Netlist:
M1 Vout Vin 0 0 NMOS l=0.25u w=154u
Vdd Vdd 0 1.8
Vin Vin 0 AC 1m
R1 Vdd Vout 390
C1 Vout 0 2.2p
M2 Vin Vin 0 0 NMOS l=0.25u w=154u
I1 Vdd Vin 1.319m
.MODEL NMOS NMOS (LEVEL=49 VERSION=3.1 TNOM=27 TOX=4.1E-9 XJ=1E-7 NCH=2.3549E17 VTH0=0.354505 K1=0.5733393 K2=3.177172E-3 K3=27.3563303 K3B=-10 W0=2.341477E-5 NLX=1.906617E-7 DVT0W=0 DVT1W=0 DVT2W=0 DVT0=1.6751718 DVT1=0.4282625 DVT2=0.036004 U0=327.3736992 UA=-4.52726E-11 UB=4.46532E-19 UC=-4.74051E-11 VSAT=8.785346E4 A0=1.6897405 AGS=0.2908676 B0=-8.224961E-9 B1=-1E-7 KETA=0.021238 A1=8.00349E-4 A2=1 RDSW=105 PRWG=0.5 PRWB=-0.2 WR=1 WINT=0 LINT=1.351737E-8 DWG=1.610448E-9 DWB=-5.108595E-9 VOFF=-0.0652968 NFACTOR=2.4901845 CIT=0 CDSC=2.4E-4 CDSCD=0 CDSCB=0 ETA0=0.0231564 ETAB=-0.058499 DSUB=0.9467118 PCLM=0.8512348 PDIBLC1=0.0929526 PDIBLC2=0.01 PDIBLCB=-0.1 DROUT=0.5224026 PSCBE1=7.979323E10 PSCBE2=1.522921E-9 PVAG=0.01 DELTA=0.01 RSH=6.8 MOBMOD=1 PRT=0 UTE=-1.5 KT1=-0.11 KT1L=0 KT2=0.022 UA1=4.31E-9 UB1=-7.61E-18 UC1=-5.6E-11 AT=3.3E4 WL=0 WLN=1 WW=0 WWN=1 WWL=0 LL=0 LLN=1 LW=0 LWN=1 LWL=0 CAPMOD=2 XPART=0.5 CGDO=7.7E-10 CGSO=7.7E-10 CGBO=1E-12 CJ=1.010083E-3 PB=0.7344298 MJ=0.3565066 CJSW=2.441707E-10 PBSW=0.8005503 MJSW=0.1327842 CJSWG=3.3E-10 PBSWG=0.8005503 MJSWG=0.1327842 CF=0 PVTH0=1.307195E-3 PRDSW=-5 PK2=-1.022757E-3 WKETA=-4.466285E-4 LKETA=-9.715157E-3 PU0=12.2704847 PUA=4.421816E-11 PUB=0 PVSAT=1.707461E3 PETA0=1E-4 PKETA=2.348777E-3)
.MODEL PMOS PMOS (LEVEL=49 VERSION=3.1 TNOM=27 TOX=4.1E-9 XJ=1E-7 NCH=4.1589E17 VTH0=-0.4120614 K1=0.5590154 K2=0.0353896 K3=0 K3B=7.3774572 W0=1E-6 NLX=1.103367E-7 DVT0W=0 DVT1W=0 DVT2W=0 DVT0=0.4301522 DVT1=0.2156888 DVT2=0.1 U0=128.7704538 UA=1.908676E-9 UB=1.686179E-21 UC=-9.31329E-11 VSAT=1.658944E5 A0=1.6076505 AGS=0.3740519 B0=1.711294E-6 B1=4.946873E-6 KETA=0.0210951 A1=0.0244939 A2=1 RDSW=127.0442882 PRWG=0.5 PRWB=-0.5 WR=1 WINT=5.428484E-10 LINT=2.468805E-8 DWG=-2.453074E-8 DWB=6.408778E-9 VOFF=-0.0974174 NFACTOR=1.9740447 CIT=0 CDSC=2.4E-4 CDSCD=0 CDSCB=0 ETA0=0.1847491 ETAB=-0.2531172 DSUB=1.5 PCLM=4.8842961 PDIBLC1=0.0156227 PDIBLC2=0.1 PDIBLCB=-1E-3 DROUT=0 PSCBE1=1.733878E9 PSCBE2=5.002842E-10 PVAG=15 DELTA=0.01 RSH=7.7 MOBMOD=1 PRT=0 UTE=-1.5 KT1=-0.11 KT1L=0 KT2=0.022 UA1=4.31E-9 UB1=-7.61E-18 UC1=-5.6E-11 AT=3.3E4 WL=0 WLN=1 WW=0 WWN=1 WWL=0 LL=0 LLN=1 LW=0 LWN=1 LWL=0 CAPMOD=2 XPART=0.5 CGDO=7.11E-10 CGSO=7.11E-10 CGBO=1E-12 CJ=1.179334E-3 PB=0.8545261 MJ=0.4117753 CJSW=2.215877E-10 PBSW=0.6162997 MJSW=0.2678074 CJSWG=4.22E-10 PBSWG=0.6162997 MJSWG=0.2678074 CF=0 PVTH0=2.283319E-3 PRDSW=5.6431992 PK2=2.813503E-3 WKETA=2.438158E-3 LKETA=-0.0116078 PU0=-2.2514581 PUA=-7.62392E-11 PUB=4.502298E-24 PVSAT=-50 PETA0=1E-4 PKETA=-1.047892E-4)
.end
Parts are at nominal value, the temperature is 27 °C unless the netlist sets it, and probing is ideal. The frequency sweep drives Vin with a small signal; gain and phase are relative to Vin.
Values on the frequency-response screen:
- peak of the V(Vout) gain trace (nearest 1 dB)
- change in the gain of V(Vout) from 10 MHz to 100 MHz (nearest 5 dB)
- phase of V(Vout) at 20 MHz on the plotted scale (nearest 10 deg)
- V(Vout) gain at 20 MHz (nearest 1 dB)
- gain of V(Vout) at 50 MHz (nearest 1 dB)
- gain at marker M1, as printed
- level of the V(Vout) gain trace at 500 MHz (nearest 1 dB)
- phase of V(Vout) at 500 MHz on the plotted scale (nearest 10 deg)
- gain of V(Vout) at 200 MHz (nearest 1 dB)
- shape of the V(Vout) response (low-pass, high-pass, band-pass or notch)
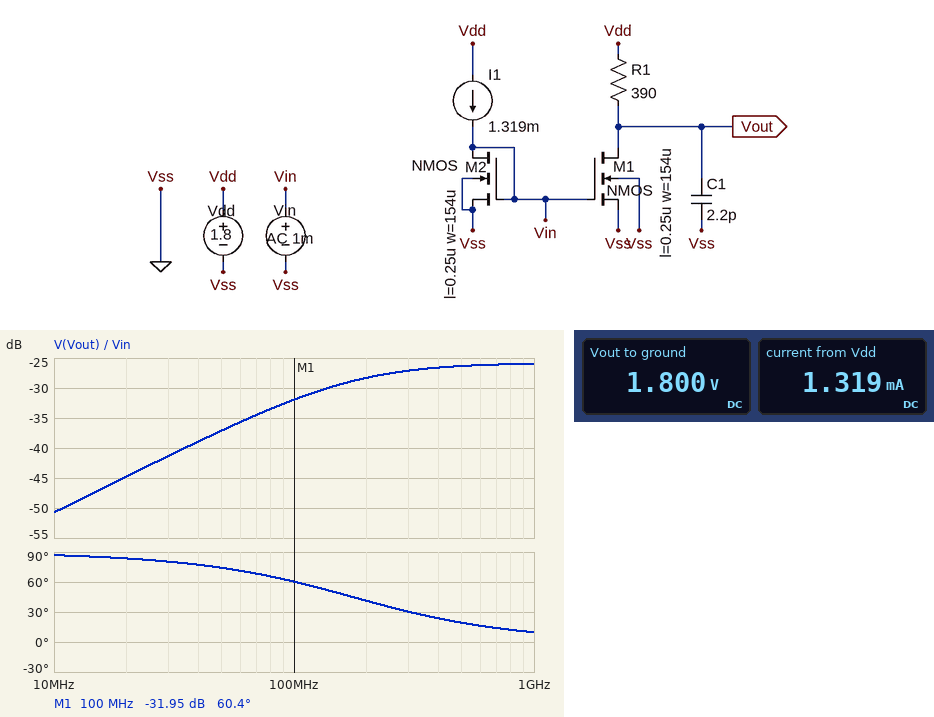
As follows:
-26 dB
20 dB
80 deg
-45 dB
-37 dB
-31.95 dB
-26 dB
20 deg
-28 dB
high-pass
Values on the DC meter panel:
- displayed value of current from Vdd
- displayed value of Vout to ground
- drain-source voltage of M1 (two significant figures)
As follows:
1.319 mA
1.800 V
1.8 V
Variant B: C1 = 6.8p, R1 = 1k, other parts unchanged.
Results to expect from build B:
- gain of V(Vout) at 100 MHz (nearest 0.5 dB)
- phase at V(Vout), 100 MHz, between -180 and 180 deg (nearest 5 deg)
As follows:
-35.5 dB
15 deg
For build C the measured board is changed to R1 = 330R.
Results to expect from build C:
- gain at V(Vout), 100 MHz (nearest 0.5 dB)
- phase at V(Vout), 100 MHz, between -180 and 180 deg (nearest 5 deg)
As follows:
-33.0 dB
65 deg
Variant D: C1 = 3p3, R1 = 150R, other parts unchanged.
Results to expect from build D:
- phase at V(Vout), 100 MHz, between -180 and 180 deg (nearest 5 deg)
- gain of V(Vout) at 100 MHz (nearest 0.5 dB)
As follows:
70 deg
-39.5 dB
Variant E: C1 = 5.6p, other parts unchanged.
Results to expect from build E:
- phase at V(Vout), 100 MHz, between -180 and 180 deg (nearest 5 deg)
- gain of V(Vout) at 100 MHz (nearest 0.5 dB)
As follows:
35 deg
-35.5 dB
